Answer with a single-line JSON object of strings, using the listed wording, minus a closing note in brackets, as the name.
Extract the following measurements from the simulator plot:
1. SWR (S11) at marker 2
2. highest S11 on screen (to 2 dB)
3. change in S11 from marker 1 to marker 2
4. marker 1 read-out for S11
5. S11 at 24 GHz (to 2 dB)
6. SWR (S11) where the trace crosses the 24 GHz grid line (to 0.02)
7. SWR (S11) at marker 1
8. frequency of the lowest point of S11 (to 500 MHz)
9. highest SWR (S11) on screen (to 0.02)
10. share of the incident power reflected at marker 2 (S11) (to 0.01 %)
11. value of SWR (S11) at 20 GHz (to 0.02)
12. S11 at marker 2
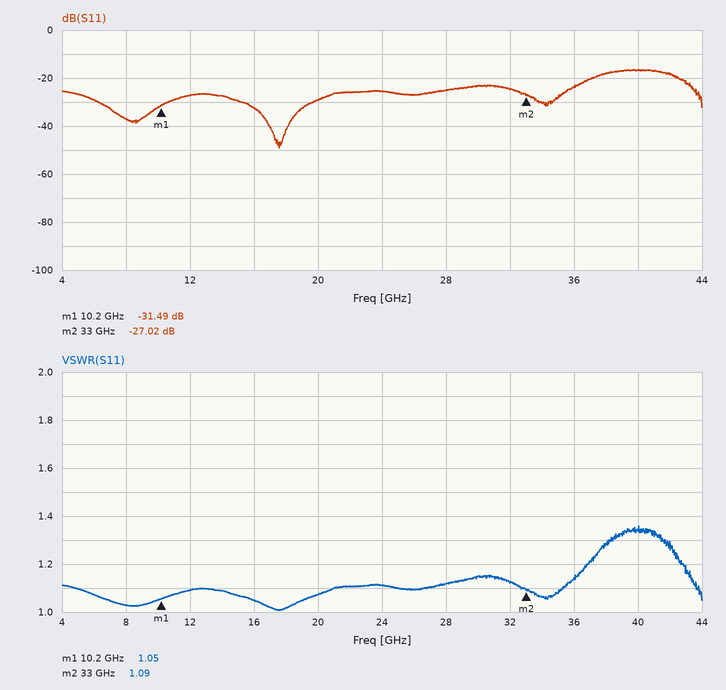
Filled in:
{"SWR (S11) at marker 2": "1.09", "highest S11 on screen": "-16 dB", "change in S11 from marker 1 to marker 2": "4.47 dB", "marker 1 read-out for S11": "-31.49 dB", "S11 at 24 GHz": "-26 dB", "SWR (S11) where the trace crosses the 24 GHz grid line": "1.12", "SWR (S11) at marker 1": "1.05", "frequency of the lowest point of S11": "17.5 GHz", "highest SWR (S11) on screen": "1.36", "share of the incident power reflected at marker 2 (S11)": "0.20 %", "value of SWR (S11) at 20 GHz": "1.08", "S11 at marker 2": "-27.02 dB"}
